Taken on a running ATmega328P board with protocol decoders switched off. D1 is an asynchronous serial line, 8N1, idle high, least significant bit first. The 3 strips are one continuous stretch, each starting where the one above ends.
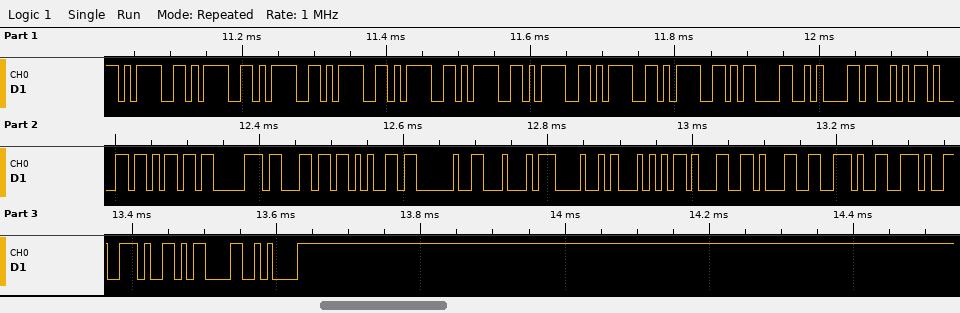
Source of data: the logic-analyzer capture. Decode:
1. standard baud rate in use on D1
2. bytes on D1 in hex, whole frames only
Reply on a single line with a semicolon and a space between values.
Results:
115200 baud; 3D 3D 3D 3D 3D 3D 3D 3D 3D 0D 0A 53 61 6D 70 6C 65 20 44 48 54 31 31 2E 2E 2E 0D 0A
